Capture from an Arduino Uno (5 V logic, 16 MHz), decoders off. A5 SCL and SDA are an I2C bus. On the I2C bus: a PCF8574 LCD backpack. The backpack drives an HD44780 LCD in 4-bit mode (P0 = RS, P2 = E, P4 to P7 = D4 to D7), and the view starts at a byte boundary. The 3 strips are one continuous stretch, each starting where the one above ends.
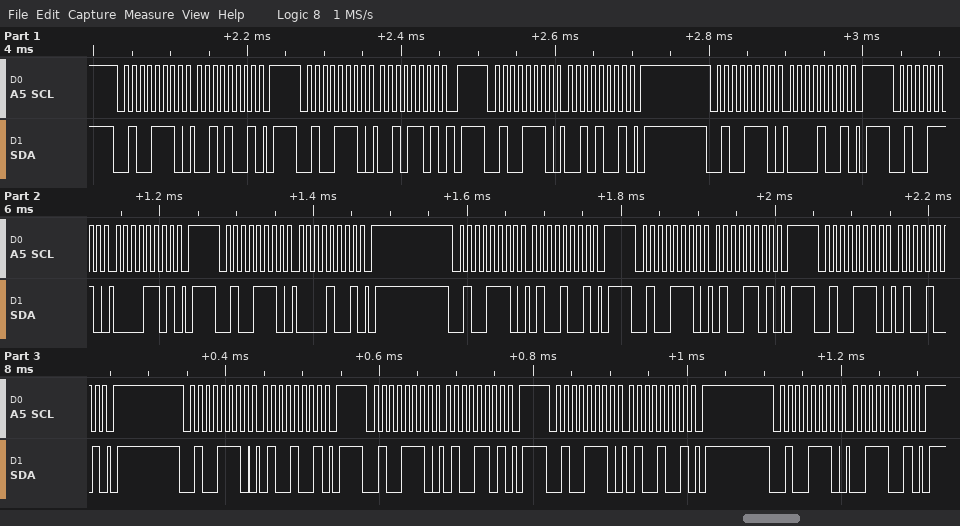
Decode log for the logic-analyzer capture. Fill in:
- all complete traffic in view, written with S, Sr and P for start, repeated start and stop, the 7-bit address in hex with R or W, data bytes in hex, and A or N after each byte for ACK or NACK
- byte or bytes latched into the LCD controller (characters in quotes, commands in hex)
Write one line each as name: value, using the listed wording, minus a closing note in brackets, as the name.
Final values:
all complete traffic in view, written with S, Sr and P for start, repeated start and stop, the 7-bit address in hex with R or W, data bytes in hex, and A or N after each byte for ACK or NACK: S 27W A 29 A P S 27W A 2D A P S 27W A 29 A P S 27W A 09 A P S 27W A 0D A P S 27W A 09 A P S 27W A 49 A P S 27W A 4D A P S 27W A 49 A P S 27W A 49 A P S 27W A 4D A P S 27W A 49 A P S 27W A 39 A P
byte or bytes latched into the LCD controller: ' ' 'D'
